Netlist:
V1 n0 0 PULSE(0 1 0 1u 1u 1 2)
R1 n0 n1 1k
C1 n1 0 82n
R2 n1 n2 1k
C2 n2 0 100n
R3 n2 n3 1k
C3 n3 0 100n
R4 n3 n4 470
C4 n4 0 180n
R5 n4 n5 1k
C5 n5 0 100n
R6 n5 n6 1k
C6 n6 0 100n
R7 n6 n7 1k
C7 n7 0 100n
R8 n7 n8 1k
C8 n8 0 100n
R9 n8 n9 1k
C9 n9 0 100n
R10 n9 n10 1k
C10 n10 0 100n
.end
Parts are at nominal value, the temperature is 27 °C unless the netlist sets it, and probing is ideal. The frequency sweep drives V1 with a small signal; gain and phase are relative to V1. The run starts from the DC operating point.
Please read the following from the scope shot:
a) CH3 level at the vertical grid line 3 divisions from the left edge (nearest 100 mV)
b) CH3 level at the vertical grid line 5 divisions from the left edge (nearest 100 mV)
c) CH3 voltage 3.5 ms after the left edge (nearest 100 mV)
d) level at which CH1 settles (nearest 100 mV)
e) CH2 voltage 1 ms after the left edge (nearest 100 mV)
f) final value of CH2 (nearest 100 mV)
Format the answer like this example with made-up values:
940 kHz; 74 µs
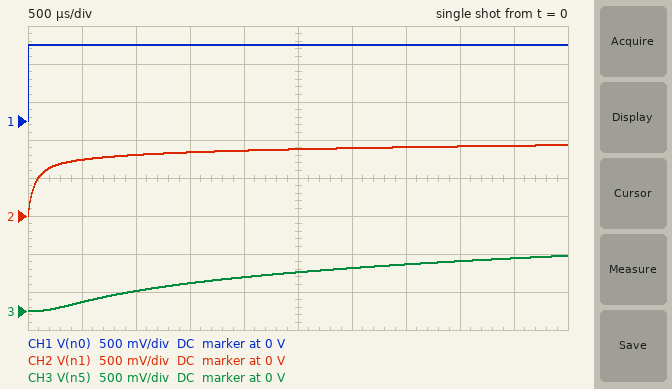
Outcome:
400 mV; 500 mV; 600 mV; 1.0 V; 800 mV; 900 mV
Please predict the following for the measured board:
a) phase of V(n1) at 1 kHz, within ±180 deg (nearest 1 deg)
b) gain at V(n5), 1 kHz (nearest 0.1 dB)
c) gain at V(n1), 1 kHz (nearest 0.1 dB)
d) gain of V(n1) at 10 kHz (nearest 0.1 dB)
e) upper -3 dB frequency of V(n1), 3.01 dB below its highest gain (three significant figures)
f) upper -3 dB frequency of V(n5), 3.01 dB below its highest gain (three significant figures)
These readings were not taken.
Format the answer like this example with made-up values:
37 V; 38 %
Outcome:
-27 deg; -25.1 dB; -4.7 dB; -15.0 dB; 327 Hz; 39.3 Hz
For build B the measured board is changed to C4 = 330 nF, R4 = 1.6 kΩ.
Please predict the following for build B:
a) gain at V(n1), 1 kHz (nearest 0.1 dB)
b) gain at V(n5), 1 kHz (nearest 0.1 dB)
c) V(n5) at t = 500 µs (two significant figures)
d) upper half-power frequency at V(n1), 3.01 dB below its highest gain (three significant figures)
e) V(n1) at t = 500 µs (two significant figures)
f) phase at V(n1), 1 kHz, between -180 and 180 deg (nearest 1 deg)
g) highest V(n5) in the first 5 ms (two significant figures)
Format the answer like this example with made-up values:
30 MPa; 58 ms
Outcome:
-4.6 dB; -31.6 dB; 56 mV; 418 Hz; 760 mV; -28 deg; 610 mV
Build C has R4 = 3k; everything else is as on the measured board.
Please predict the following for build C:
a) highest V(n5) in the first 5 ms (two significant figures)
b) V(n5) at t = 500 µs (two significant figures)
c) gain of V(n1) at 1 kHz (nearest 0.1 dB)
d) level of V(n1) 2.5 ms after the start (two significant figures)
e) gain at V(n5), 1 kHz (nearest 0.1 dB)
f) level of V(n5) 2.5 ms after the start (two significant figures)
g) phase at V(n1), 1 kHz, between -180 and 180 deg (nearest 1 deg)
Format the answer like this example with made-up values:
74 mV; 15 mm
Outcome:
580 mV; 56 mV; -4.8 dB; 900 mV; -31.6 dB; 370 mV; -29 deg
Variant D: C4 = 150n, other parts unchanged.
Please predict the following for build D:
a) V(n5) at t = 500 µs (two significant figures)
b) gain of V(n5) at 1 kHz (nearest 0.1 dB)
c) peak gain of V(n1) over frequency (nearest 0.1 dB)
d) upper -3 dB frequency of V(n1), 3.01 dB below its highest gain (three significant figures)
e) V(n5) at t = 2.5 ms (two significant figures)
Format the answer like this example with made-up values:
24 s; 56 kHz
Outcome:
130 mV; -24.5 dB; 0 dB; 339 Hz; 520 mV
